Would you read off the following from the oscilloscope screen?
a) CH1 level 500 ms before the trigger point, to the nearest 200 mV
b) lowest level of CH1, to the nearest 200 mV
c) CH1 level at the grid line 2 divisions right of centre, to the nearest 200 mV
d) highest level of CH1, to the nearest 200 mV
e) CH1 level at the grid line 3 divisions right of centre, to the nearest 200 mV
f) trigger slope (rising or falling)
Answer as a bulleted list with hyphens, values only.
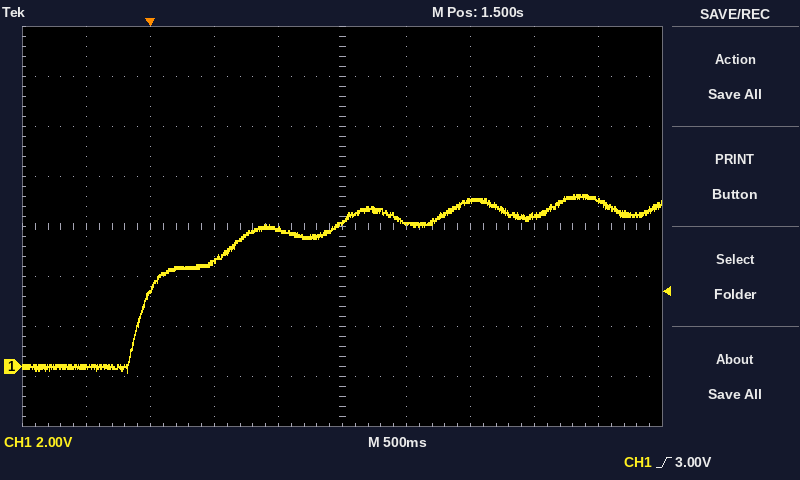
- 0.0 V
- -200 mV
- 6.6 V
- 6.8 V
- 6.0 V
- rising
